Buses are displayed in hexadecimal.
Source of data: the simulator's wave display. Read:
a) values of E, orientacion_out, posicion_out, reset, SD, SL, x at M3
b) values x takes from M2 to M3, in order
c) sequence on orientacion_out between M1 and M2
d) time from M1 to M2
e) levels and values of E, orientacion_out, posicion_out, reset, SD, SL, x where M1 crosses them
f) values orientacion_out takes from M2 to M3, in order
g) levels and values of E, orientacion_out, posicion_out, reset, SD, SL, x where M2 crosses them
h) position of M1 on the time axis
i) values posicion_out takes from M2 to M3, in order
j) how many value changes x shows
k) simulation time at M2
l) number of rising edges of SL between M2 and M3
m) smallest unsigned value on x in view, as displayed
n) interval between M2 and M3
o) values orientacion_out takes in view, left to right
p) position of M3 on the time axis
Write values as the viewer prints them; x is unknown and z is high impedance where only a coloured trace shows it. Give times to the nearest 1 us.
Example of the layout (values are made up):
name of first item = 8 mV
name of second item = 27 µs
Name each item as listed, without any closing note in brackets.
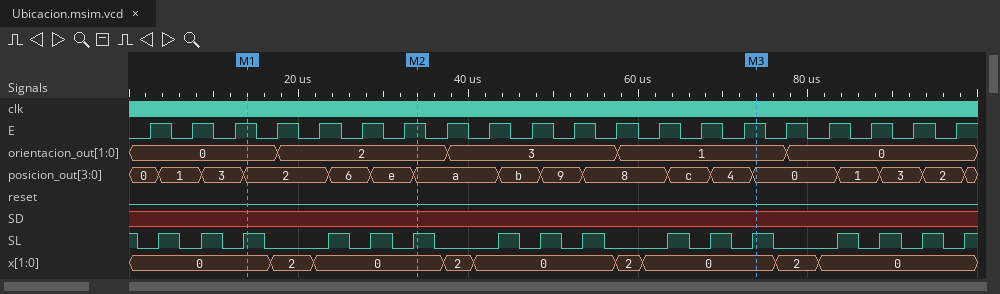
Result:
values of E, orientacion_out, posicion_out, reset, SD, SL, x at M3 = E=1, orientacion_out=1, posicion_out=0, reset=0, SD=x, SL=1, x=0
values x takes from M2 to M3, in order = 0, 2, 0, 2, 0
sequence on orientacion_out between M1 and M2 = 0, 2
time from M1 to M2 = 20 us
levels and values of E, orientacion_out, posicion_out, reset, SD, SL, x where M1 crosses them = E=1, orientacion_out=0, posicion_out=2, reset=0, SD=x, SL=1, x=0
values orientacion_out takes from M2 to M3, in order = 2, 3, 1
levels and values of E, orientacion_out, posicion_out, reset, SD, SL, x where M2 crosses them = E=1, orientacion_out=2, posicion_out=a, reset=0, SD=x, SL=1, x=0
position of M1 on the time axis = 14 us
values posicion_out takes from M2 to M3, in order = a, b, 9, 8, c, 4, 0
how many value changes x shows = 8
simulation time at M2 = 34 us
number of rising edges of SL between M2 and M3 = 6
smallest unsigned value on x in view, as displayed = 0
interval between M2 and M3 = 40 us
values orientacion_out takes in view, left to right = 0, 2, 3, 1, 0
position of M3 on the time axis = 74 us
